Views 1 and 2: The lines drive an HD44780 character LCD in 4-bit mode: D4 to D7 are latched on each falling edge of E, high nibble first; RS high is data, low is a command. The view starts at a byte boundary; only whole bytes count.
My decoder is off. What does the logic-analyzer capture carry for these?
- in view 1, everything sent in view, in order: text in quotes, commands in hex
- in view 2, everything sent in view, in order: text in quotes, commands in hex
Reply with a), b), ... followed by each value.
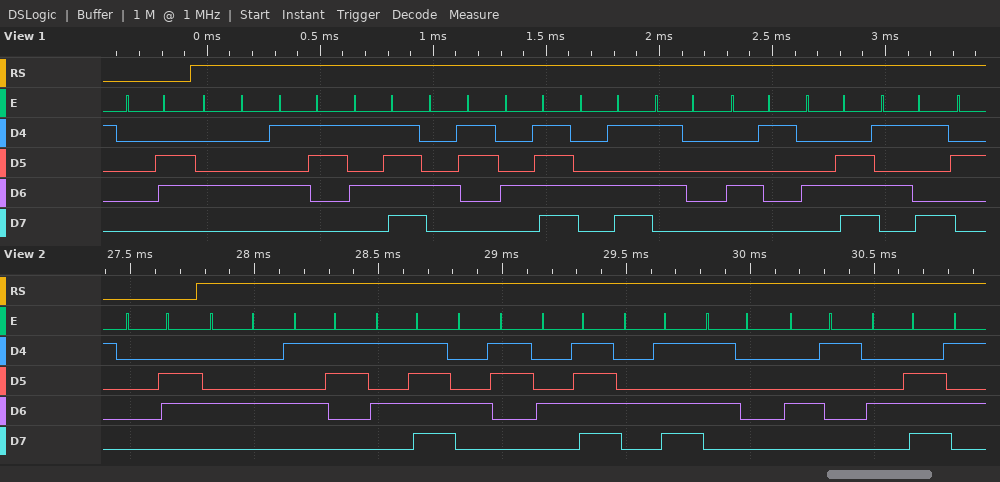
a) 0x06 "DS_COMPANY"
b) 0x06 "DS_COMPAN"
